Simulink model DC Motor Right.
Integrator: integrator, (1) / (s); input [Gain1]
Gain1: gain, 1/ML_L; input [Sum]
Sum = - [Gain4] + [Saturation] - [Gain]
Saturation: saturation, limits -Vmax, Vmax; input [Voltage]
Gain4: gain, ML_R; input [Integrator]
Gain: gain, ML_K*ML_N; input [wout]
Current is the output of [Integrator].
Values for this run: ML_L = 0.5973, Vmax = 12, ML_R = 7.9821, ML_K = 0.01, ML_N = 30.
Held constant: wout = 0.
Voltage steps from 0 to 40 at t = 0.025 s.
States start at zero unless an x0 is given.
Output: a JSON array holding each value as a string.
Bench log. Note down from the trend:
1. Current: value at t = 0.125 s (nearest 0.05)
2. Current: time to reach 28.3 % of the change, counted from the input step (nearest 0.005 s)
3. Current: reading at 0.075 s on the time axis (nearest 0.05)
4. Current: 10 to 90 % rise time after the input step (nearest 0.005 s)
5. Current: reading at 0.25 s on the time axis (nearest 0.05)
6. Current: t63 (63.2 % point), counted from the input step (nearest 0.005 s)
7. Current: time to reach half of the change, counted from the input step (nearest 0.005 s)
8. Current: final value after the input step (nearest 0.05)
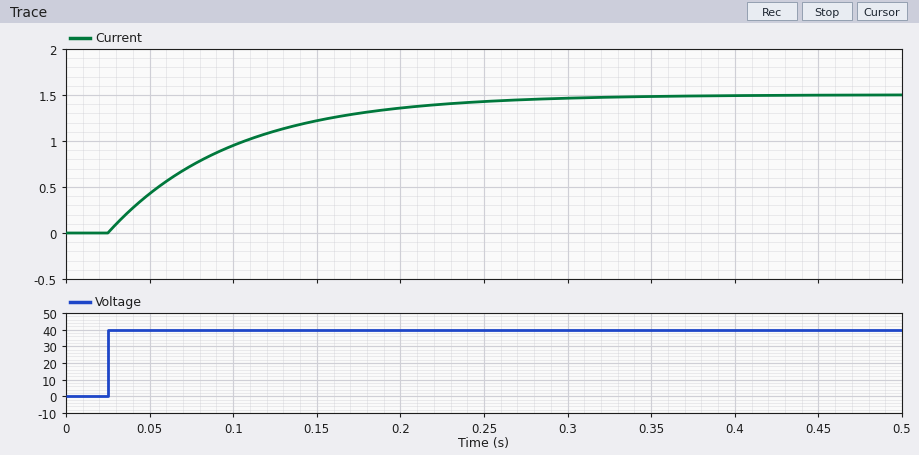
["1.10", "0.025 s", "0.75", "0.165 s", "1.45", "0.075 s", "0.050 s", "1.50"]
